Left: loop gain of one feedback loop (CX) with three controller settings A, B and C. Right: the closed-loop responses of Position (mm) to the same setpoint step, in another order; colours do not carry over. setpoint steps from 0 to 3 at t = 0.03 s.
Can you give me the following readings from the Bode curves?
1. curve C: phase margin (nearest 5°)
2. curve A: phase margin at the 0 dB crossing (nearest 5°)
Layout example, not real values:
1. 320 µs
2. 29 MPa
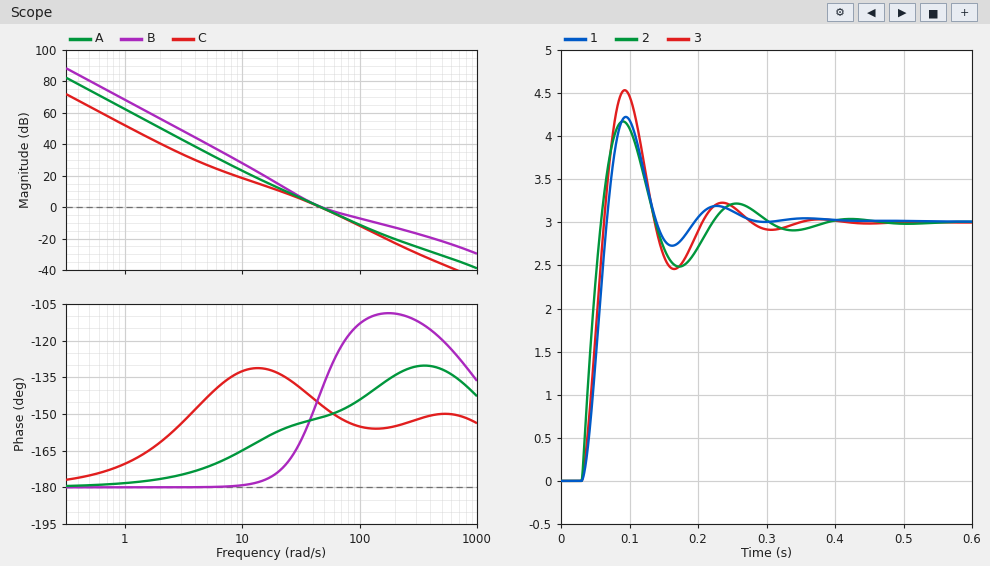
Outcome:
1. 35°
2. 30°
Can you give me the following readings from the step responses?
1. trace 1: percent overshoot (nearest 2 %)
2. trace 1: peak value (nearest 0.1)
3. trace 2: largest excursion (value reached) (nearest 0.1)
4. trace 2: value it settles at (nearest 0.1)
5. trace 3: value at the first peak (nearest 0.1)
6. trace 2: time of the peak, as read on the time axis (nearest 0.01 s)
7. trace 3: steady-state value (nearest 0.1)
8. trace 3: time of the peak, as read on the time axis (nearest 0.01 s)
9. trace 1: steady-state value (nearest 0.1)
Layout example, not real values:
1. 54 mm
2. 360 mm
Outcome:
1. 40 %
2. 4.2
3. 4.2
4. 3.0
5. 4.5
6. 0.09 s
7. 3.0
8. 0.09 s
9. 3.0
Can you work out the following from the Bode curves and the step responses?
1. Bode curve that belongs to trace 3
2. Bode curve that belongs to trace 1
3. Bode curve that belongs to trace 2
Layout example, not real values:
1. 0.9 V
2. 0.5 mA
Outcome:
1. A
2. C
3. B
